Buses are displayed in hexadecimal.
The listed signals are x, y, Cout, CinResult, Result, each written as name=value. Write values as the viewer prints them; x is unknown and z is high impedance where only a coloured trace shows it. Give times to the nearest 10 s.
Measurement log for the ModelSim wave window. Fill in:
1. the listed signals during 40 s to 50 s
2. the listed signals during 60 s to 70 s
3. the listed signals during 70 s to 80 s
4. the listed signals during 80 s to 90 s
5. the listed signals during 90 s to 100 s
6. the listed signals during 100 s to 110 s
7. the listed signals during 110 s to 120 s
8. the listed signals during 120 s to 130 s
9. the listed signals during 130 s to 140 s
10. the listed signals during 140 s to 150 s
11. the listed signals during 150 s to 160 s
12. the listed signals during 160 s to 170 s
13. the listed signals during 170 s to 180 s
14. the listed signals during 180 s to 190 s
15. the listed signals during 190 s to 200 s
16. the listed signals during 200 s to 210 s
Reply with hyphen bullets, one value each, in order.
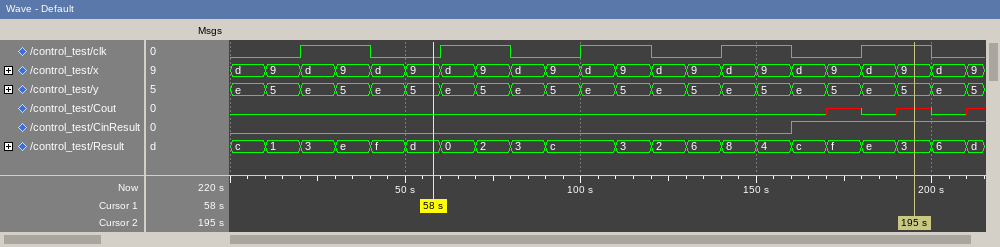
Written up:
- x=d, y=e, Cout=0, CinResult=0, Result=f
- x=d, y=e, Cout=0, CinResult=0, Result=0
- x=9, y=5, Cout=0, CinResult=0, Result=2
- x=d, y=e, Cout=0, CinResult=0, Result=3
- x=9, y=5, Cout=0, CinResult=0, Result=c
- x=d, y=e, Cout=0, CinResult=0, Result=c
- x=9, y=5, Cout=0, CinResult=0, Result=3
- x=d, y=e, Cout=0, CinResult=0, Result=2
- x=9, y=5, Cout=0, CinResult=0, Result=6
- x=d, y=e, Cout=0, CinResult=0, Result=8
- x=9, y=5, Cout=0, CinResult=0, Result=4
- x=d, y=e, Cout=0, CinResult=1, Result=c
- x=9, y=5, Cout=x, CinResult=1, Result=f
- x=d, y=e, Cout=0, CinResult=1, Result=e
- x=9, y=5, Cout=x, CinResult=1, Result=3
- x=d, y=e, Cout=0, CinResult=1, Result=6
